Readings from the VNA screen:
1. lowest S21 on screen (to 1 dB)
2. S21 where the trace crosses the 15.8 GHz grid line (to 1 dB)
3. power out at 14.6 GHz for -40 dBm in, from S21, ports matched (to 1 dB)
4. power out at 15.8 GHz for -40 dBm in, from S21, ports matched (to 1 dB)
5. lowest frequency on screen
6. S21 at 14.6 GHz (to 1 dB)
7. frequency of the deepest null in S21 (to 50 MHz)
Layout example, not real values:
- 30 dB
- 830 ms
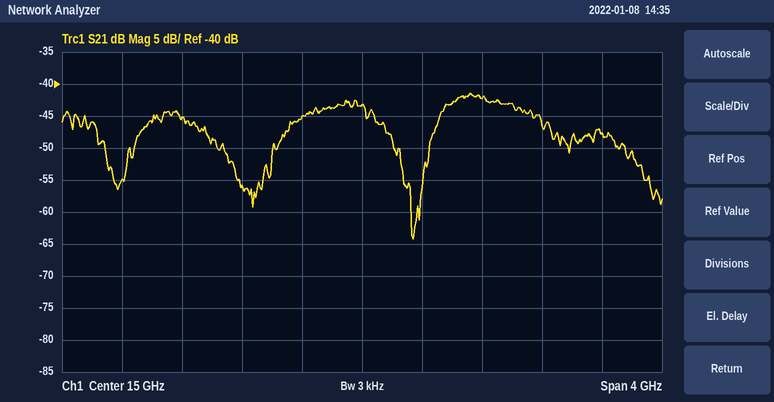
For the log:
- -64 dB
- -42 dB
- -85 dBm
- -82 dBm
- 13 GHz
- -45 dB
- 15.35 GHz
